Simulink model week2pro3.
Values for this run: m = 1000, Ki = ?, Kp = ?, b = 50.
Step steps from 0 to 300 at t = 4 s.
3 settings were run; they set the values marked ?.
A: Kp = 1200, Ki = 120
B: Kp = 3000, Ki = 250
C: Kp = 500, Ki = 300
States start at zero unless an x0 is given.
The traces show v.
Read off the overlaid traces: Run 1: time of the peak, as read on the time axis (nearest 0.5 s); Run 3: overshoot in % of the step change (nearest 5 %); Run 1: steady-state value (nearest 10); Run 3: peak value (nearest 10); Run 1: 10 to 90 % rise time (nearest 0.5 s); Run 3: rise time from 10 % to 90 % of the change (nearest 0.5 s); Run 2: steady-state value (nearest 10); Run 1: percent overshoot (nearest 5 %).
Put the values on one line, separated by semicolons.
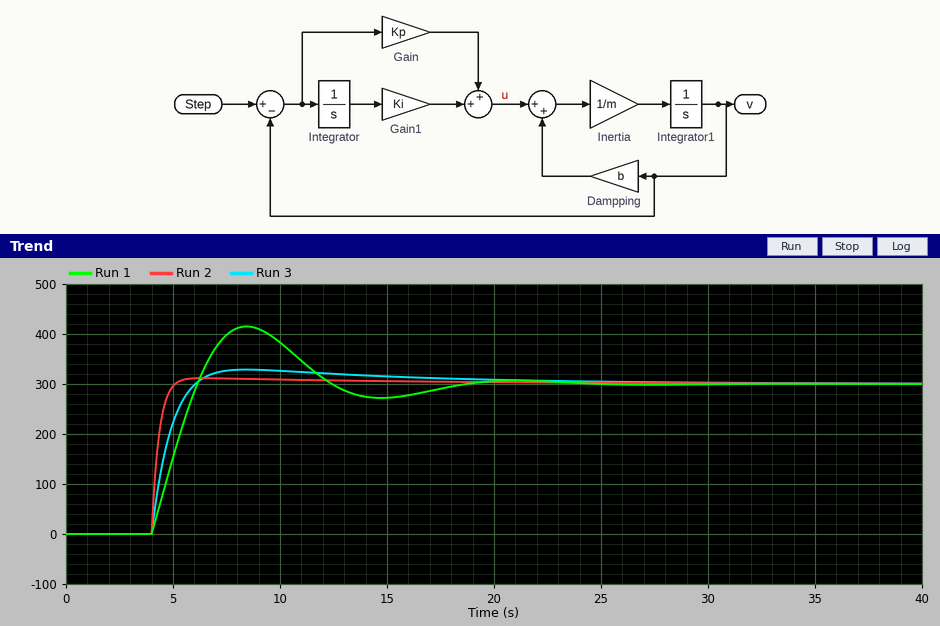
8.5 s; 10 %; 300; 330; 1.5 s; 1.5 s; 300; 40 %
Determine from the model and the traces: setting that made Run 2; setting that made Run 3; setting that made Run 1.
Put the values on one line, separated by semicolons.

B; A; C
